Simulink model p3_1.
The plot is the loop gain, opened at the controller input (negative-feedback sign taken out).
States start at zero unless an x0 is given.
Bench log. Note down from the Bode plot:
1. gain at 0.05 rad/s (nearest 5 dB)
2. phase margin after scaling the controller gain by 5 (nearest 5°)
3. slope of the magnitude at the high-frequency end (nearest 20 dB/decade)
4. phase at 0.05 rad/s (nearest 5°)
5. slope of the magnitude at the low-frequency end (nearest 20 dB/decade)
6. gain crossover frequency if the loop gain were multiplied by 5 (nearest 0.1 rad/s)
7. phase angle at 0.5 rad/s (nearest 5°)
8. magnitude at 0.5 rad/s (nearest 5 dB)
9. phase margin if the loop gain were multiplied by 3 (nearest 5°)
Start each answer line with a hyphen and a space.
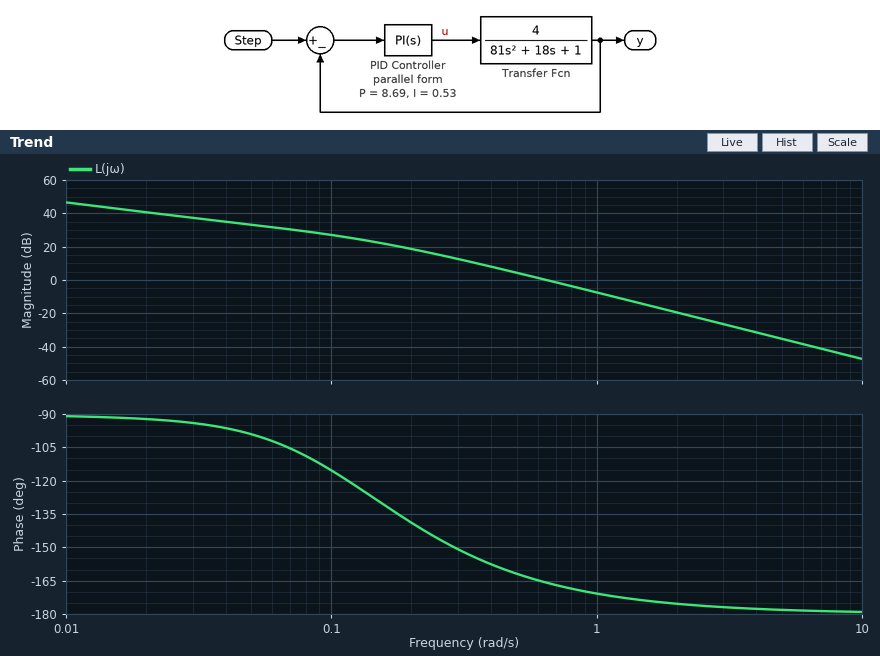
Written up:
- 35 dB
- 5°
- -40 dB/decade
- -100°
- -20 dB/decade
- 1.5 rad/s
- -160°
- 5 dB
- 10°
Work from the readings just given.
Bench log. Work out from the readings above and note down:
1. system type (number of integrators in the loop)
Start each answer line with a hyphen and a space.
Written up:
- 1
